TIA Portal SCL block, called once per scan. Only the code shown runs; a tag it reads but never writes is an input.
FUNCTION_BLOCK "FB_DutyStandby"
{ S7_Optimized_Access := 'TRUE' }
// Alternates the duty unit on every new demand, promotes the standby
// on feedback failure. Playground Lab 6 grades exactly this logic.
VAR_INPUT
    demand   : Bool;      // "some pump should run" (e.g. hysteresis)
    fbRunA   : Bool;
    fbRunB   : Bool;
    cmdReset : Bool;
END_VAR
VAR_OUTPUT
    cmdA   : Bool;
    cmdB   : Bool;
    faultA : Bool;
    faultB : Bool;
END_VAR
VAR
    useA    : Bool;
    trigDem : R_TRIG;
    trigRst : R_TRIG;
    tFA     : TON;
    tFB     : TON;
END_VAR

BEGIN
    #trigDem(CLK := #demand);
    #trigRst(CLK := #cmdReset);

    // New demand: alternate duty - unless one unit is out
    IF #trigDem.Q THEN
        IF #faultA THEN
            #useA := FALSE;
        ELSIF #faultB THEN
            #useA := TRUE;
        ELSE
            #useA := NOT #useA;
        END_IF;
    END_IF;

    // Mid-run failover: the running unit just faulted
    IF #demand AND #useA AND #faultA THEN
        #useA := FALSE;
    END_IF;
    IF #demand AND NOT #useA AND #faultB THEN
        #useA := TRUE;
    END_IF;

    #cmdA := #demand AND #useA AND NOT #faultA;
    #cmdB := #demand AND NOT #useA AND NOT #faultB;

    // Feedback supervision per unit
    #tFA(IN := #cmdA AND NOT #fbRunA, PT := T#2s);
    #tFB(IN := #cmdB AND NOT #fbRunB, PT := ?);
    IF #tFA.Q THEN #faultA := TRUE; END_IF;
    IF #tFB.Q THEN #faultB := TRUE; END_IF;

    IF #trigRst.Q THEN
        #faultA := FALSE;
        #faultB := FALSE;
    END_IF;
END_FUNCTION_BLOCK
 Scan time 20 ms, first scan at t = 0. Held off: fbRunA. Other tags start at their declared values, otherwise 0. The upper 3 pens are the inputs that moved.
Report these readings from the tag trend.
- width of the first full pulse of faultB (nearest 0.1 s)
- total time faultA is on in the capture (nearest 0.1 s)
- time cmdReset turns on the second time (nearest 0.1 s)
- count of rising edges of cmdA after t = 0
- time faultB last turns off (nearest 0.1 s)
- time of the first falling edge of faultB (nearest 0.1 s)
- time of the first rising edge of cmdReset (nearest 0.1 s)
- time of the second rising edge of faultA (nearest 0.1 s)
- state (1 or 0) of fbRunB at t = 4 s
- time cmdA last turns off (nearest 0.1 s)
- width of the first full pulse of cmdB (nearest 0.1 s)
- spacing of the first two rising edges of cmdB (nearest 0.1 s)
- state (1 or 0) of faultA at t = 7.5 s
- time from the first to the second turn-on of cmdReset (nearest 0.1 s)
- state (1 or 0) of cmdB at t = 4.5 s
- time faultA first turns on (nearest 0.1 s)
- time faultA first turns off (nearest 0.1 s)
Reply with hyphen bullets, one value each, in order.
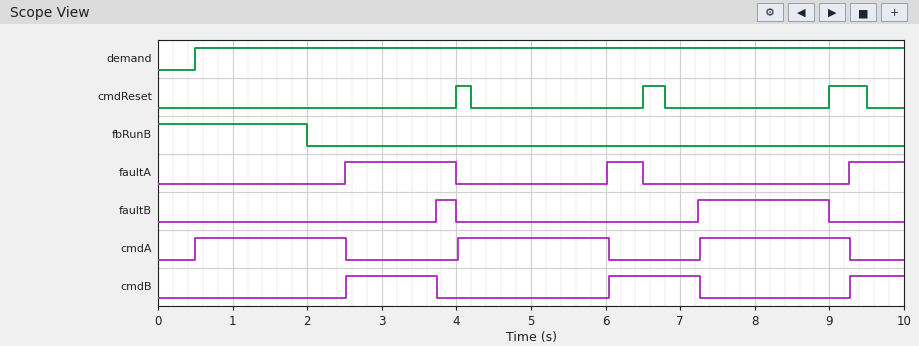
- 0.3 s
- 2.7 s
- 6.5 s
- 3
- 9.0 s
- 4.0 s
- 4.0 s
- 6.0 s
- 0
- 9.3 s
- 1.2 s
- 3.5 s
- 0
- 2.5 s
- 0
- 2.5 s
- 4.0 s
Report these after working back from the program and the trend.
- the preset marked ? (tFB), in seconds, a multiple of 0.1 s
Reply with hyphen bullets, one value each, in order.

- 1.2 s
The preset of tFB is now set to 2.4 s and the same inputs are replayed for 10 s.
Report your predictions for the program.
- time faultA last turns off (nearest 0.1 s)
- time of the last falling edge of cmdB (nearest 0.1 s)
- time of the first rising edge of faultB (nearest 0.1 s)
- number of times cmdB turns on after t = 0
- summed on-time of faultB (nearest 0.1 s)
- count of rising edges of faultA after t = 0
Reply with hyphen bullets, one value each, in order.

- 9.0 s
- 9.4 s
- 4.9 s
- 2
- 2.2 s
- 2
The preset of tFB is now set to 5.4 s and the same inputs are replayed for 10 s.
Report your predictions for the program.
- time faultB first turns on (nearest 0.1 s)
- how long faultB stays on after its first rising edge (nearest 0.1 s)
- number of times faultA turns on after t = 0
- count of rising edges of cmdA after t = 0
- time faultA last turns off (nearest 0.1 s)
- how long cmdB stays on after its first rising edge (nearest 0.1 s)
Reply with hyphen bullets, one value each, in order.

- 7.9 s
- 1.1 s
- 2
- 2
- 4.0 s
- 5.4 s
